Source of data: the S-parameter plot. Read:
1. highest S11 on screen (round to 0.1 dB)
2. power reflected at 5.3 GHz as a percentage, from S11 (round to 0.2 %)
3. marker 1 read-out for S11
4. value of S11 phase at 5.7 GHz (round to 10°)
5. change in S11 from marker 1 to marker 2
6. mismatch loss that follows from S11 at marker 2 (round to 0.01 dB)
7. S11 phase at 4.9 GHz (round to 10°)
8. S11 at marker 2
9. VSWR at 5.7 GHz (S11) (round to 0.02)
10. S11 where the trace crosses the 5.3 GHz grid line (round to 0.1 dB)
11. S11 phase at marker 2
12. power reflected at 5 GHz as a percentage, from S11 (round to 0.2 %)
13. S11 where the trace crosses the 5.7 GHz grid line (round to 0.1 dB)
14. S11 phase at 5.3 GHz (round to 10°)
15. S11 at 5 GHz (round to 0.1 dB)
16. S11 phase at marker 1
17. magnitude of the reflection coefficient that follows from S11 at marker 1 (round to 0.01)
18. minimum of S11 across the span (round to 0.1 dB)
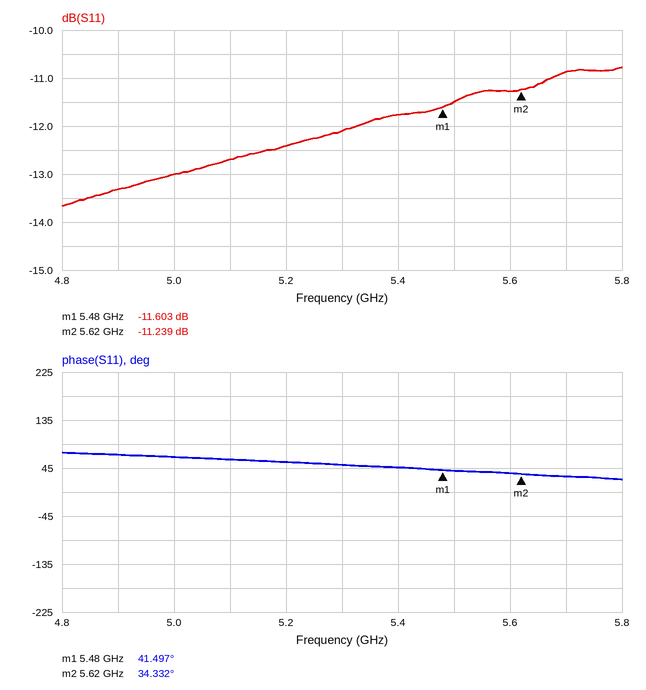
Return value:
-10.8 dB
6.2 %
-11.603 dB
30°
0.364 dB
0.34 dB
70°
-11.239 dB
1.80
-12.1 dB
34.332°
5.0 %
-10.9 dB
50°
-13.0 dB
41.497°
0.26
-13.7 dB
